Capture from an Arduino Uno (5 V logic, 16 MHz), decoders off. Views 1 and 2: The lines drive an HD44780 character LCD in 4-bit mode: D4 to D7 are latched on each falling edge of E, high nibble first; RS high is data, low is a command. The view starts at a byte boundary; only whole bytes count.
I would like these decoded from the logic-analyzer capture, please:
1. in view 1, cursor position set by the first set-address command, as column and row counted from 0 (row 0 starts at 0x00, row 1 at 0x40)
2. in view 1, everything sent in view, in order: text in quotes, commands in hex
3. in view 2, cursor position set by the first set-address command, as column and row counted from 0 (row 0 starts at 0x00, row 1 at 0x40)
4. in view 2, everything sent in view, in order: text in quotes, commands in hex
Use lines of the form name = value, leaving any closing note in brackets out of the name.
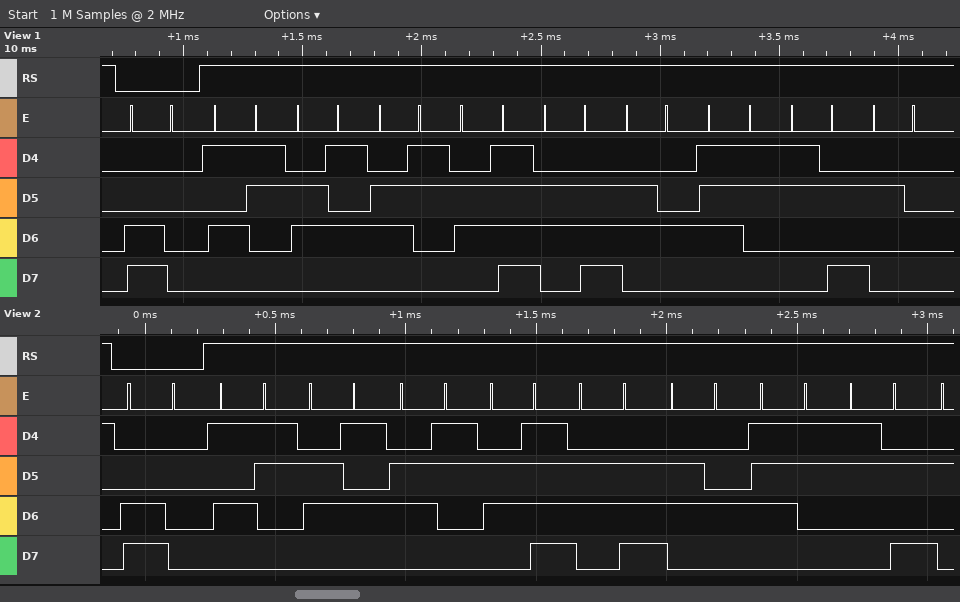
in view 1, cursor position set by the first set-address command, as column and row counted from 0 = column 0, row 1
in view 1, everything sent in view, in order: text in quotes, commands in hex = 0xC0 "Seconds: "
in view 2, cursor position set by the first set-address command, as column and row counted from 0 = column 0, row 1
in view 2, everything sent in view, in order: text in quotes, commands in hex = 0xC0 "Seconds:"
